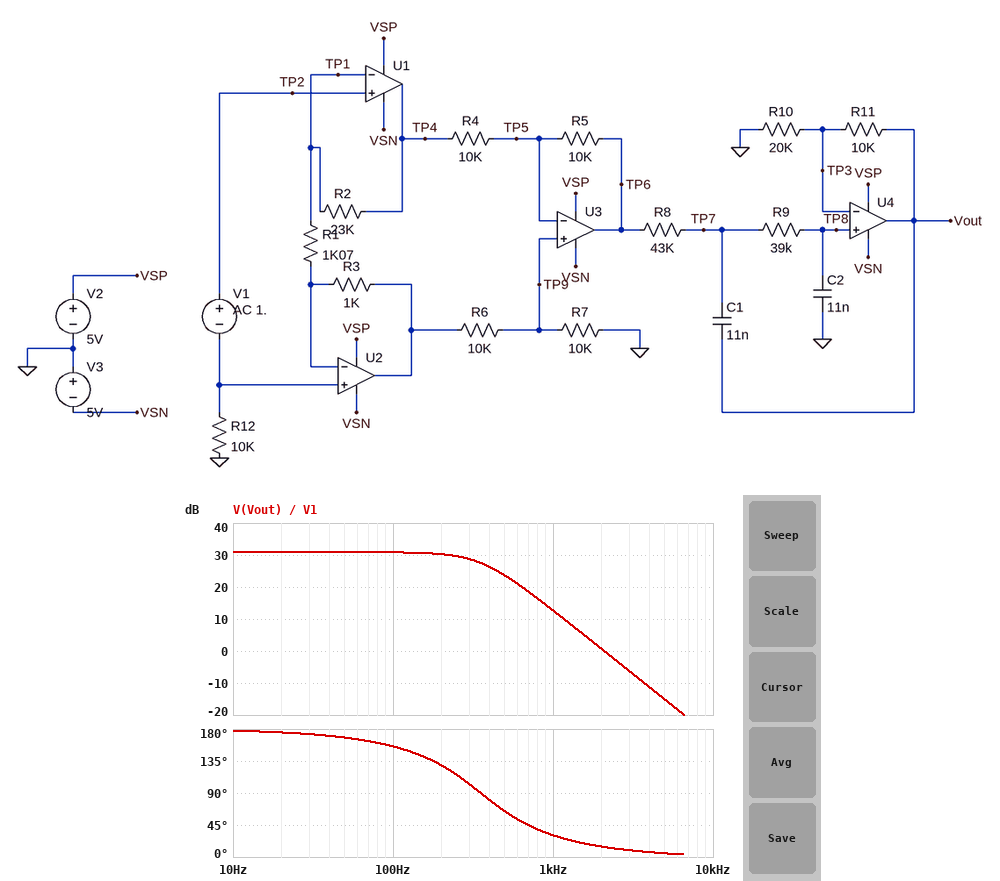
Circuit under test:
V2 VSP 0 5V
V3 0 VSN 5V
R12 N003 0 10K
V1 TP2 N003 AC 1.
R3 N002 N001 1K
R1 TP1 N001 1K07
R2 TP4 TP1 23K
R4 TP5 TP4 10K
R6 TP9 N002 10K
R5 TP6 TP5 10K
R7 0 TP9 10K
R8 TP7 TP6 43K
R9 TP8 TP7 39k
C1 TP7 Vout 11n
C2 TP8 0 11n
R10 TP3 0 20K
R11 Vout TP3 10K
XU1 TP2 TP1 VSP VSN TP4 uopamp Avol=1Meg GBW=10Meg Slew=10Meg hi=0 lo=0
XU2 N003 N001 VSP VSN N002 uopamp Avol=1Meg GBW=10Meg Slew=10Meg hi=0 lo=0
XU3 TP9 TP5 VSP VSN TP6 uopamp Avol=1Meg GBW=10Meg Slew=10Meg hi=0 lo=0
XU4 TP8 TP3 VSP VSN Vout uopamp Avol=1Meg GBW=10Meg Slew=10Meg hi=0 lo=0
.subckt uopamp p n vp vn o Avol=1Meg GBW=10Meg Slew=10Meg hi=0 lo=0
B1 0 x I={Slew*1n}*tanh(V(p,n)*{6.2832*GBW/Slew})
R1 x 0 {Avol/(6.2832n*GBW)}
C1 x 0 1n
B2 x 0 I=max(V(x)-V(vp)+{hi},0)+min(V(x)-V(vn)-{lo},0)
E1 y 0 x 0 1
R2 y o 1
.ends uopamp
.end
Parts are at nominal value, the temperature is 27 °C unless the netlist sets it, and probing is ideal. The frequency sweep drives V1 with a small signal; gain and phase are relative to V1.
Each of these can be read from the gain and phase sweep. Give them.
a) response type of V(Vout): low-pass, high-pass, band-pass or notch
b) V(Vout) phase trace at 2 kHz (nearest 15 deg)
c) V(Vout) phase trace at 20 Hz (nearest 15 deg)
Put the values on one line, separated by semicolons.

low-pass; 15 deg; 180 deg
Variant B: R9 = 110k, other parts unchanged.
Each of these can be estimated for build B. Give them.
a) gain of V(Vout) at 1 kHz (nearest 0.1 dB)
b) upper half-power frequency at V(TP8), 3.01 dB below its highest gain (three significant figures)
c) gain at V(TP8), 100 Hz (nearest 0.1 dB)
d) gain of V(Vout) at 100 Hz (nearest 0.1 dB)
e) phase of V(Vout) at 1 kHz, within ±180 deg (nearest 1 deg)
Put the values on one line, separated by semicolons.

3.5 dB; 144 Hz; 25.9 dB; 29.4 dB; 23 deg
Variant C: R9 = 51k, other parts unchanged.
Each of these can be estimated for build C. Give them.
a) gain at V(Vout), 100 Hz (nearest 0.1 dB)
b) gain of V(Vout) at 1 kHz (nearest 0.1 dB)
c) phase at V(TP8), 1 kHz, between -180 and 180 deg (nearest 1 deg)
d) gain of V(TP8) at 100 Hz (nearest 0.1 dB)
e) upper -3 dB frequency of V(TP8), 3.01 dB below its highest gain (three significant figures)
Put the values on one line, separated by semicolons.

30.7 dB; 10.3 dB; 28 deg; 27.2 dB; 280 Hz
